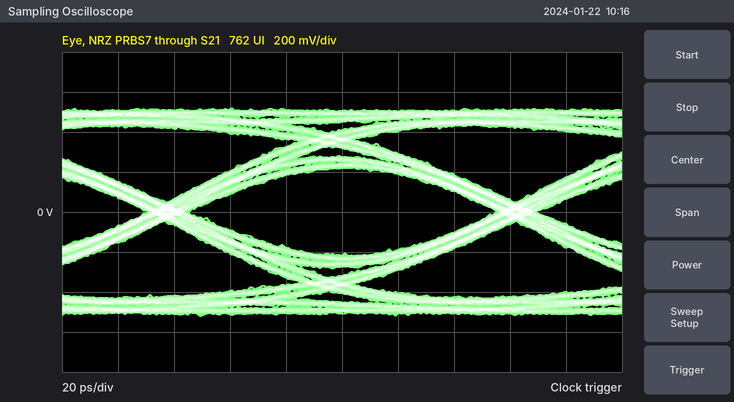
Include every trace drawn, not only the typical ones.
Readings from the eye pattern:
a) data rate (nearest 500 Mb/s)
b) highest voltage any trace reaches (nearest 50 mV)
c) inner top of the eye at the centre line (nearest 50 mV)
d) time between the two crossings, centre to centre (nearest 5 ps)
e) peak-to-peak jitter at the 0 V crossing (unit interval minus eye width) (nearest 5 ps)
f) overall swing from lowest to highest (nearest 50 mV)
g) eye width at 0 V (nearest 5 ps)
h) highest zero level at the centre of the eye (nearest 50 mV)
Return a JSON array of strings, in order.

["8.0 Gb/s", "500 mV", "200 mV", "125 ps", "15 ps", "1.05 V", "110 ps", "-200 mV"]
